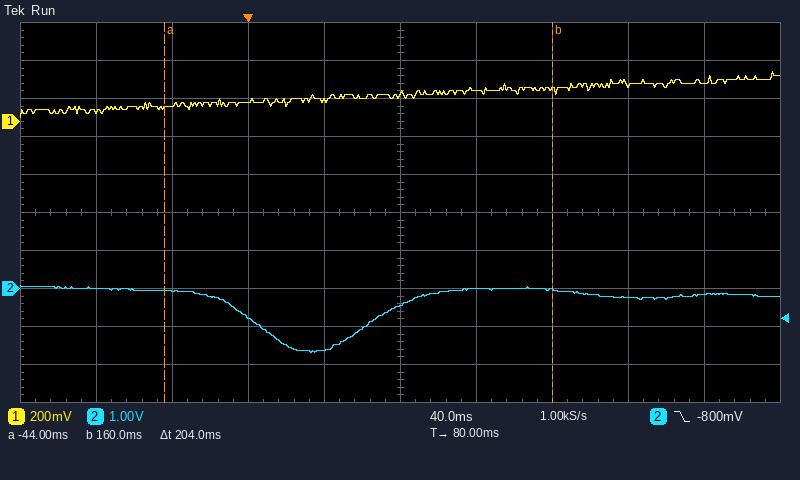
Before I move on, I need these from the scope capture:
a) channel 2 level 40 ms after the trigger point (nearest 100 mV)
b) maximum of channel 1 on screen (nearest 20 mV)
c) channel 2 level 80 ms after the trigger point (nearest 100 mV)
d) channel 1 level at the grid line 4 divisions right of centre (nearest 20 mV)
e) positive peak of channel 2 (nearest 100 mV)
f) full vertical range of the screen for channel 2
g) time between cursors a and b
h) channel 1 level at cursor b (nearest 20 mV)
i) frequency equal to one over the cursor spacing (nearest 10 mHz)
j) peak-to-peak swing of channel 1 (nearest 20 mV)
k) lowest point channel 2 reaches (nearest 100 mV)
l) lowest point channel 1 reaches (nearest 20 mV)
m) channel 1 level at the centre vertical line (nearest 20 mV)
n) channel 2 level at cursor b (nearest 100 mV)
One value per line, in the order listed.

-1.6 V
260 mV
-400 mV
200 mV
100 mV
10 V
204 ms
160 mV
4.90 Hz
240 mV
-1.7 V
20 mV
140 mV
0.0 V
